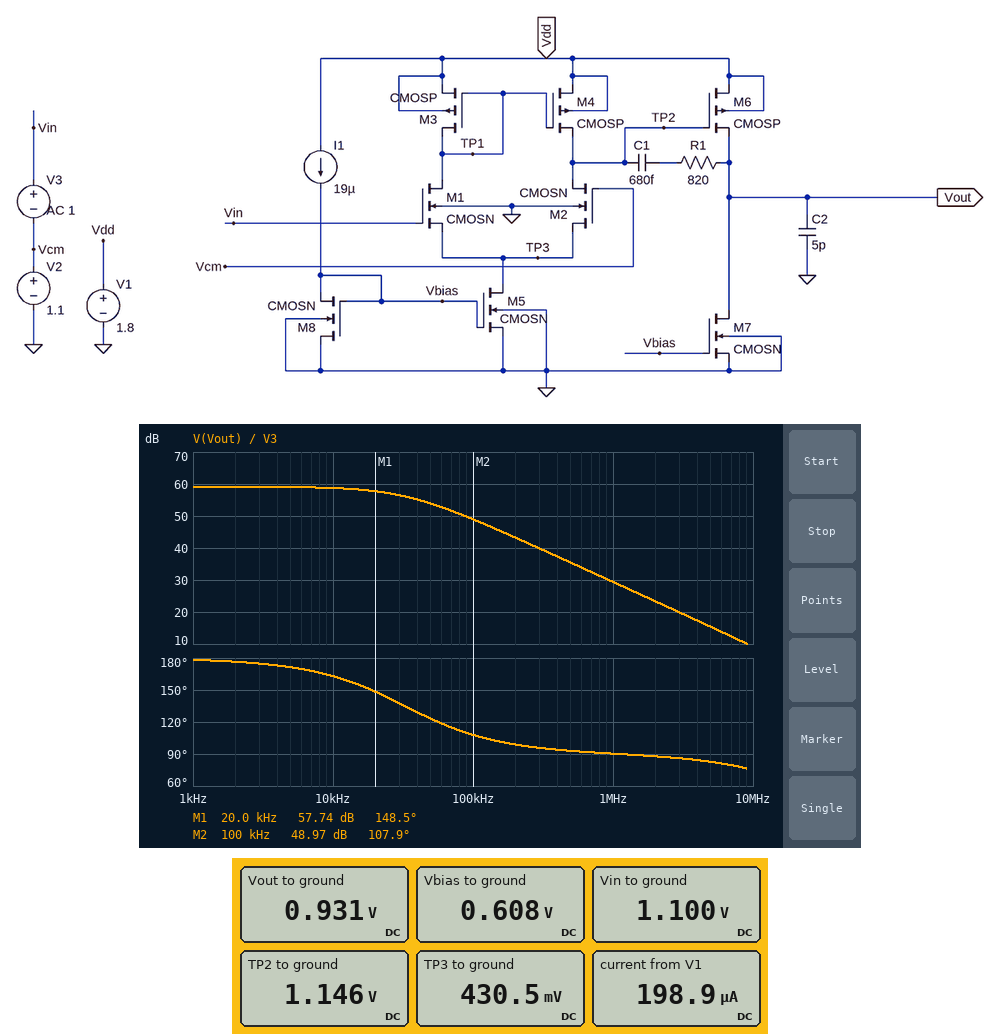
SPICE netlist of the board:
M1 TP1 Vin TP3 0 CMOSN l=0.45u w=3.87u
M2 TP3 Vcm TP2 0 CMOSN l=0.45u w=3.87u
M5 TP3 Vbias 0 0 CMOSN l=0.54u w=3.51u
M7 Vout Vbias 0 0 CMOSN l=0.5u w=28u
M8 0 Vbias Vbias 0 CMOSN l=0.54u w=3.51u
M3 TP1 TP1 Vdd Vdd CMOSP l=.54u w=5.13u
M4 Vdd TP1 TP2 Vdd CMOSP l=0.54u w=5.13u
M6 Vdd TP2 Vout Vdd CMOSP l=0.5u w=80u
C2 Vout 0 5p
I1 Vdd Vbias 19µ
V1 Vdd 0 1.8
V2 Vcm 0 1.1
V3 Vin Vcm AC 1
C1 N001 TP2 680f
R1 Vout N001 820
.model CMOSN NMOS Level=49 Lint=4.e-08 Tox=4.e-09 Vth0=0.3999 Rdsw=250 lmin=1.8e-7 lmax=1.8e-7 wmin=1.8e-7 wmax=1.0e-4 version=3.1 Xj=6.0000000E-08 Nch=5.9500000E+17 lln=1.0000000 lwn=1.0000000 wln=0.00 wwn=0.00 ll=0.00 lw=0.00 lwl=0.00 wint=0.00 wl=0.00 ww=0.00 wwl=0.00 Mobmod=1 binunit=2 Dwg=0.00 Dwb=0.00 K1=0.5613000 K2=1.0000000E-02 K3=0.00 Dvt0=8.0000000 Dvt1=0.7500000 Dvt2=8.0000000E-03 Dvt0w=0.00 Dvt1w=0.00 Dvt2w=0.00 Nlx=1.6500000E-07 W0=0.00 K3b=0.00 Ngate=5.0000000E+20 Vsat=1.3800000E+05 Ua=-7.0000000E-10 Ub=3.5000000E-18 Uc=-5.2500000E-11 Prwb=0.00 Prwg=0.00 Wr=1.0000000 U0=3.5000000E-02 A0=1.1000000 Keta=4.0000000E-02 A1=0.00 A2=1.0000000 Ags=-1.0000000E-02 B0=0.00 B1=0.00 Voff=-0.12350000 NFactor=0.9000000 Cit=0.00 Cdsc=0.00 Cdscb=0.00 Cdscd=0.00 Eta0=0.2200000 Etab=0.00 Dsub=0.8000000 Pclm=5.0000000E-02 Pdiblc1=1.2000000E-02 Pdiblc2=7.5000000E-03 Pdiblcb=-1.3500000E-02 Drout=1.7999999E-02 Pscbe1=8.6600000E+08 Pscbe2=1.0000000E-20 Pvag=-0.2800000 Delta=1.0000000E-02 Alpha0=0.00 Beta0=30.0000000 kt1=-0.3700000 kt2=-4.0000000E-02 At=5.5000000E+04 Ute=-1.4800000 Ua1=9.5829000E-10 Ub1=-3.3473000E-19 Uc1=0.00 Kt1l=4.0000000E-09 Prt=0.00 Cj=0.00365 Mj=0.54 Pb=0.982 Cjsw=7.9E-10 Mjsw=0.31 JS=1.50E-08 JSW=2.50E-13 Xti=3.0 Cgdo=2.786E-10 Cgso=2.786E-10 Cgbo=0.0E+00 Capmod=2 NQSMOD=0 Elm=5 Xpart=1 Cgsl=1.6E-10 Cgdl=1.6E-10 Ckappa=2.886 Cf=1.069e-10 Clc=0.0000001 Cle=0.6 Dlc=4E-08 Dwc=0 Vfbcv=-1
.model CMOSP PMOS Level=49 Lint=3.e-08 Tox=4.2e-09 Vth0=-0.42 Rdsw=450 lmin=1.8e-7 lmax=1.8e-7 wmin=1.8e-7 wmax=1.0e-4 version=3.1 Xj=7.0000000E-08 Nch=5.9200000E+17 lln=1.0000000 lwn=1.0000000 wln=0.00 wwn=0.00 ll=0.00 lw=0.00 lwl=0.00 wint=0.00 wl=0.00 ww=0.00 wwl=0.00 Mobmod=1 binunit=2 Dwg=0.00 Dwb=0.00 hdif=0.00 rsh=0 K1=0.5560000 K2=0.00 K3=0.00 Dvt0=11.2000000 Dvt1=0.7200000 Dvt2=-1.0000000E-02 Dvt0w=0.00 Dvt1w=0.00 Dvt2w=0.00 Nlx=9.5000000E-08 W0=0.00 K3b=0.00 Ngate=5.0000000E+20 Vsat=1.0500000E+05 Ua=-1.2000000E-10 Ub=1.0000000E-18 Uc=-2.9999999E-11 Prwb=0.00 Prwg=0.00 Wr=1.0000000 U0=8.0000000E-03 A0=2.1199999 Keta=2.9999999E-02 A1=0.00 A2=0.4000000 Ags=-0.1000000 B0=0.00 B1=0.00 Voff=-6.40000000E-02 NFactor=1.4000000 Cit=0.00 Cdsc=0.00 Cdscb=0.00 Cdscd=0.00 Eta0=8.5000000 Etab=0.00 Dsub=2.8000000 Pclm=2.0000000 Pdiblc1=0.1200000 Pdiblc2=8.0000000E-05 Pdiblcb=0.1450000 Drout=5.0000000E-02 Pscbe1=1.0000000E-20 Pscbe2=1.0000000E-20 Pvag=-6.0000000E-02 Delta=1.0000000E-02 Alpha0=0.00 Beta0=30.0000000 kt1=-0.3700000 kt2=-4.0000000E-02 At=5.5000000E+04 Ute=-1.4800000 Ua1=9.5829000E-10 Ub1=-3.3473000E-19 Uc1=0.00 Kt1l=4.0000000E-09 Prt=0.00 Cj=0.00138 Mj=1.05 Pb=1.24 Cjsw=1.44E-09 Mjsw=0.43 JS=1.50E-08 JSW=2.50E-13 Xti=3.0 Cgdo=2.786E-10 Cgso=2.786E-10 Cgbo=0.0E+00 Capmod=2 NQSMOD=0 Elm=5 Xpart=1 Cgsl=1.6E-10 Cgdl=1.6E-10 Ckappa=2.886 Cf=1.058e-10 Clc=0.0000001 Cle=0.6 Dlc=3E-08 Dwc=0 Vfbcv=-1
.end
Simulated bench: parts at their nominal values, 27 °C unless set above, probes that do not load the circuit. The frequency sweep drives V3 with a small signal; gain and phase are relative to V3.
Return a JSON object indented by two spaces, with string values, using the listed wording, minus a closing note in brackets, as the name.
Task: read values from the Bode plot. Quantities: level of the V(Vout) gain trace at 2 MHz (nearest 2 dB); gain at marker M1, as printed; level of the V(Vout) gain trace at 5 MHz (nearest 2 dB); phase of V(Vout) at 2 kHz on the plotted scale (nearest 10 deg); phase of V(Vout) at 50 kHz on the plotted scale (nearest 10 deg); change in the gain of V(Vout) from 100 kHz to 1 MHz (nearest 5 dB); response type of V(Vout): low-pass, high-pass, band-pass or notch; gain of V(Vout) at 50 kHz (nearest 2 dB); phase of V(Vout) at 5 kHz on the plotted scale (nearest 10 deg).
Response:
{
  "level of the V(Vout) gain trace at 2 MHz": "24 dB",
  "gain at marker M1, as printed": "57.74 dB",
  "level of the V(Vout) gain trace at 5 MHz": "16 dB",
  "phase of V(Vout) at 2 kHz on the plotted scale": "180 deg",
  "phase of V(Vout) at 50 kHz on the plotted scale": "120 deg",
  "change in the gain of V(Vout) from 100 kHz to 1 MHz": "-20 dB",
  "response type of V(Vout): low-pass, high-pass, band-pass or notch": "low-pass",
  "gain of V(Vout) at 50 kHz": "54 dB",
  "phase of V(Vout) at 5 kHz on the plotted scale": "170 deg"
}
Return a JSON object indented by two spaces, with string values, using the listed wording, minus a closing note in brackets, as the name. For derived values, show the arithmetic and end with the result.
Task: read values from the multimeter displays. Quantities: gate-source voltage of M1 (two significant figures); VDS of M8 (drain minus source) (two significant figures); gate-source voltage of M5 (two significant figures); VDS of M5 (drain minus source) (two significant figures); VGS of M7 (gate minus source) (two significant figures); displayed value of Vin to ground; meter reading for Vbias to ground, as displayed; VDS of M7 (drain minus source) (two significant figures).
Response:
{
  "gate-source voltage of M1": "1.1 V - 430.5 mV = 670 mV",
  "VDS of M8 (drain minus source)": "0 V - 608 mV = -610 mV",
  "gate-source voltage of M5": "608 mV = 610 mV",
  "VDS of M5 (drain minus source)": "430.5 mV = 430 mV",
  "VGS of M7 (gate minus source)": "608 mV = 610 mV",
  "displayed value of Vin to ground": "1.100 V",
  "meter reading for Vbias to ground, as displayed": "0.608 V",
  "VDS of M7 (drain minus source)": "931 mV = 930 mV"
}
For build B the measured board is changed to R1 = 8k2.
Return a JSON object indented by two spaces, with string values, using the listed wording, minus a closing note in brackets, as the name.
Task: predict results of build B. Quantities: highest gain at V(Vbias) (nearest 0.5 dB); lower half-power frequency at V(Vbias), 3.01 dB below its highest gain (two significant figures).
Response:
{
  "highest gain at V(Vbias)": "-36.0 dB",
  "lower half-power frequency at V(Vbias), 3.01 dB below its highest gain": "78 kHz"
}
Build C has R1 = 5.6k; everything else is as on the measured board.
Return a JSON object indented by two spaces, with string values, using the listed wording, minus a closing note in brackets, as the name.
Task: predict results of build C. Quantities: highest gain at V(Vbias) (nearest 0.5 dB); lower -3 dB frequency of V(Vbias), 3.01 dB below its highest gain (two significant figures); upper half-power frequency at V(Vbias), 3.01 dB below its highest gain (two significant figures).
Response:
{
  "highest gain at V(Vbias)": "-38.0 dB",
  "lower -3 dB frequency of V(Vbias), 3.01 dB below its highest gain": "34 kHz",
  "upper half-power frequency at V(Vbias), 3.01 dB below its highest gain": "140 MHz"
}
